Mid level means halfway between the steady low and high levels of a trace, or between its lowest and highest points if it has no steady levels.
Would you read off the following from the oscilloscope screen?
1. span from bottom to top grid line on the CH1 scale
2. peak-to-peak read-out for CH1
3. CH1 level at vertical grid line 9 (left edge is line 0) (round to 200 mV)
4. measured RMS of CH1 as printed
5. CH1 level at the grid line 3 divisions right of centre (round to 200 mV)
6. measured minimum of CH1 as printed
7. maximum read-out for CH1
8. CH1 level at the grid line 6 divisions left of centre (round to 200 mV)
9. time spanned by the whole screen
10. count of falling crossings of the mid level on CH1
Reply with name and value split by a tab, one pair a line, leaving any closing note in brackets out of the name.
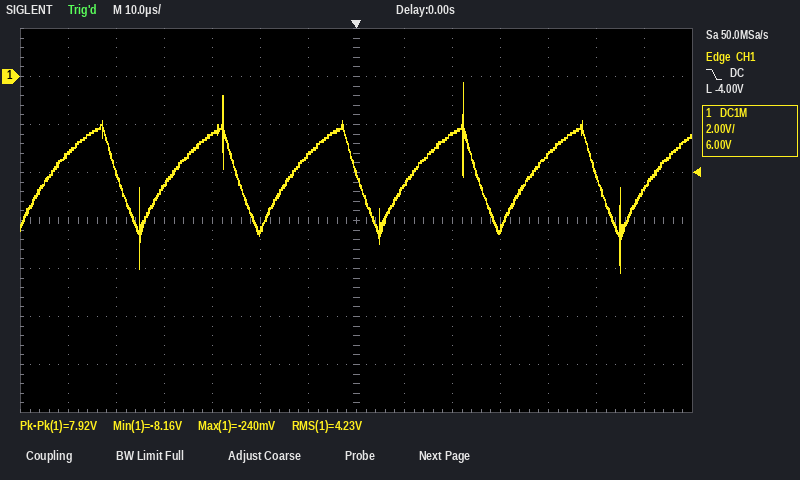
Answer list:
span from bottom to top grid line on the CH1 scale	16 V
peak-to-peak read-out for CH1	7.92 V
CH1 level at vertical grid line 9 (left edge is line 0)	-2.4 V
measured RMS of CH1 as printed	4.23 V
CH1 level at the grid line 3 divisions right of centre	-6.4 V
measured minimum of CH1 as printed	-8.16 V
maximum read-out for CH1	-240 mV
CH1 level at the grid line 6 divisions left of centre	-3.2 V
time spanned by the whole screen	140 µs
count of falling crossings of the mid level on CH1	5
